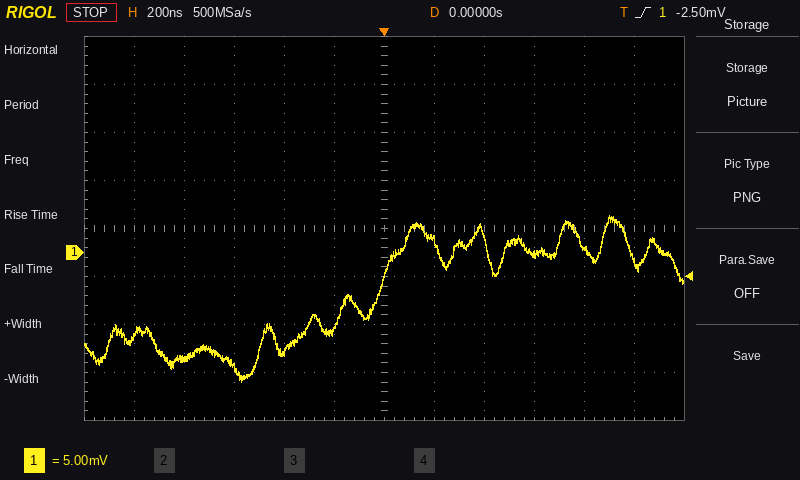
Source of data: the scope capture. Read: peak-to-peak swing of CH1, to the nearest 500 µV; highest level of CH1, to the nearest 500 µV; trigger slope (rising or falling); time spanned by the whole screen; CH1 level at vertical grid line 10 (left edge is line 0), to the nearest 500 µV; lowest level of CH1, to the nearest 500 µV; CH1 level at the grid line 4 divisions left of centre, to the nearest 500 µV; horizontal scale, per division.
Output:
17.5 mV
4.0 mV
rising
2.4 µs
500 µV
-13.5 mV
-11.0 mV
200 ns
